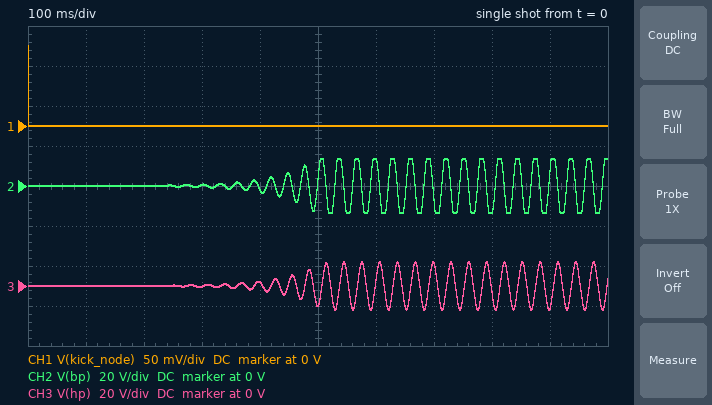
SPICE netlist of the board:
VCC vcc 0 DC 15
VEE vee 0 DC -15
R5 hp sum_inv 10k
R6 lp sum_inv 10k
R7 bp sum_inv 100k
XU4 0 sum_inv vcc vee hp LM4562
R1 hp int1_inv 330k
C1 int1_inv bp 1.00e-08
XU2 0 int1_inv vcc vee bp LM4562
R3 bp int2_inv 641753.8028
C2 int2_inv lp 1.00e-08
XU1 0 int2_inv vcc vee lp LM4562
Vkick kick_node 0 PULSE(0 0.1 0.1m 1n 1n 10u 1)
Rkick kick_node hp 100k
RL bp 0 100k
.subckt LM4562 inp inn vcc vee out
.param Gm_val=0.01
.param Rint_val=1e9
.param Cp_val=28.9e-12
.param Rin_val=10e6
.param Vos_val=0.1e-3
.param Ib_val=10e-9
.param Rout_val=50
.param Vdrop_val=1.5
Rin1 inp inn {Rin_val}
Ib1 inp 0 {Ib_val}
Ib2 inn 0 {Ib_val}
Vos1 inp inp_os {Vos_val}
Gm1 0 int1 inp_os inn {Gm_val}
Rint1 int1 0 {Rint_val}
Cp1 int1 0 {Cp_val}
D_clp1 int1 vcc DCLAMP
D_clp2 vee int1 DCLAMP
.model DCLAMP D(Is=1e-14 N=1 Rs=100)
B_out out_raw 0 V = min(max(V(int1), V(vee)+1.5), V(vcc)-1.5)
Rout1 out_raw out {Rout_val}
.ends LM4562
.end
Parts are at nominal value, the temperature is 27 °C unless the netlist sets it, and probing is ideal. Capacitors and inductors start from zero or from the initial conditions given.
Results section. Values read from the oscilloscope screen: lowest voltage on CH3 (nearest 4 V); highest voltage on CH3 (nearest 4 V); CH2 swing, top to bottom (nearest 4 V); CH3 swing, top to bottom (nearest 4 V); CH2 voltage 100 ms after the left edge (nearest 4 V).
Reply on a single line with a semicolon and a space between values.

-12 V; 12 V; 28 V; 24 V; 0 V
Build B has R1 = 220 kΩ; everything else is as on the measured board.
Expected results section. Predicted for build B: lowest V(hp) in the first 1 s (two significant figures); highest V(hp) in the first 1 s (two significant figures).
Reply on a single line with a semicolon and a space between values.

-9.9 V; 9.9 V
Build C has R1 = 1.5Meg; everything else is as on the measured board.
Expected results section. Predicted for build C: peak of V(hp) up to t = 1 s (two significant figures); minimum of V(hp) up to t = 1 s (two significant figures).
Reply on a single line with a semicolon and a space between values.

460 mV; -480 mV
